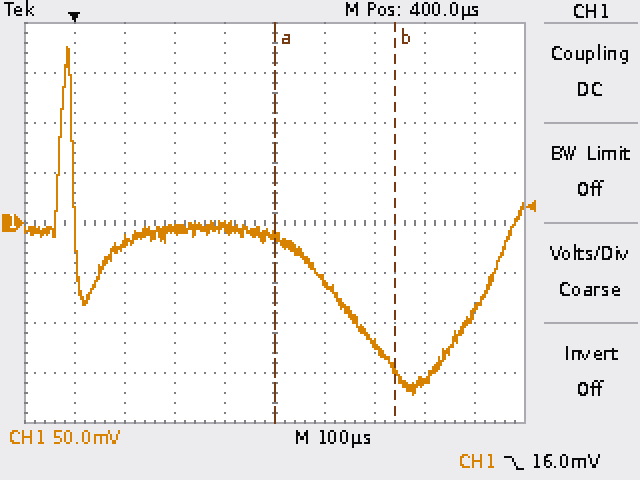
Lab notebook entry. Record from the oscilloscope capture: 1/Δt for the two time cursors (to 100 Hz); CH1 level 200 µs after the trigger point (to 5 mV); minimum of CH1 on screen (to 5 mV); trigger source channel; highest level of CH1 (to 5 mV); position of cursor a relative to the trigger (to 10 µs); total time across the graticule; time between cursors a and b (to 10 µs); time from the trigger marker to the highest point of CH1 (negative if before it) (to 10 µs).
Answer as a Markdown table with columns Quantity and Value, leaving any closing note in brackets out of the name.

| Quantity | Value |
|---|---|
| 1/Δt for the two time cursors | 4.2 kHz |
| CH1 level 200 µs after the trigger point | -5 mV |
| minimum of CH1 on screen | -170 mV |
| trigger source channel | CH1 |
| highest level of CH1 | 175 mV |
| position of cursor a relative to the trigger | +400 µs |
| total time across the graticule | 1 ms |
| time between cursors a and b | 240 µs |
| time from the trigger marker to the highest point of CH1 (negative if before it) | -10 µs |
